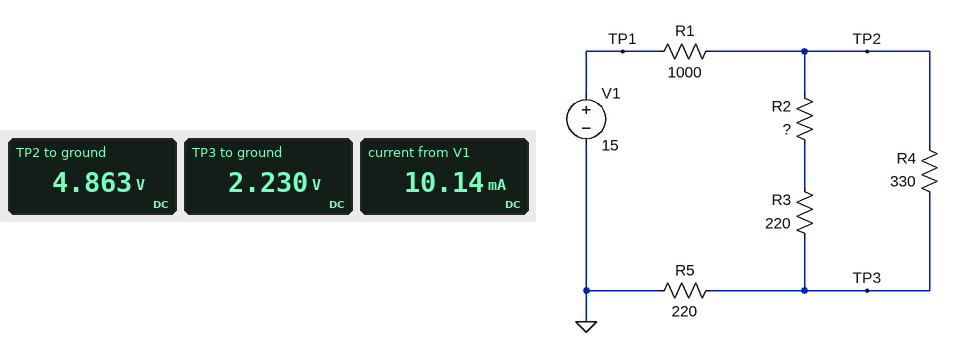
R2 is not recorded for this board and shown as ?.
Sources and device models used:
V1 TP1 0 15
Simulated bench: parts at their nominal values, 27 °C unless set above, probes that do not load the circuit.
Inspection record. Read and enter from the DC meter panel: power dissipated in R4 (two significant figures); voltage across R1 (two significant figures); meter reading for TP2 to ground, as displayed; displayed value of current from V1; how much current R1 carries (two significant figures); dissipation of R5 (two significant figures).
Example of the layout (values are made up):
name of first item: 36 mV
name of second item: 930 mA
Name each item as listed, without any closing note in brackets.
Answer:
power dissipated in R4: 21 mW
voltage across R1: 10 V
meter reading for TP2 to ground, as displayed: 4.863 V
displayed value of current from V1: 10.14 mA
how much current R1 carries: 10 mA
dissipation of R5: 23 mW
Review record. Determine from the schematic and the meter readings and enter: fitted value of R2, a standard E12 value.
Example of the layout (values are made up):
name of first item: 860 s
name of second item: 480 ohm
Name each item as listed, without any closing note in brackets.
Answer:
fitted value of R2, a standard E12 value: 1 kΩ
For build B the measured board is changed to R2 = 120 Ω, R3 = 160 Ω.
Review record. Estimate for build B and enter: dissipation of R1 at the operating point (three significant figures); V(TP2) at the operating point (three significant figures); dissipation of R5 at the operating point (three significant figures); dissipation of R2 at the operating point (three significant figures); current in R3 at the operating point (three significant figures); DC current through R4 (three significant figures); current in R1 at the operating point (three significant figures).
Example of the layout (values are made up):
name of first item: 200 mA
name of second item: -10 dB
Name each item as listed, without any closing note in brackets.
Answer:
dissipation of R1 at the operating point: 120 mW
V(TP2) at the operating point: 4.06 V
dissipation of R5 at the operating point: 26.3 mW
dissipation of R2 at the operating point: 4.20 mW
current in R3 at the operating point: 5.92 mA
DC current through R4: 5.02 mA
current in R1 at the operating point: 10.9 mA
